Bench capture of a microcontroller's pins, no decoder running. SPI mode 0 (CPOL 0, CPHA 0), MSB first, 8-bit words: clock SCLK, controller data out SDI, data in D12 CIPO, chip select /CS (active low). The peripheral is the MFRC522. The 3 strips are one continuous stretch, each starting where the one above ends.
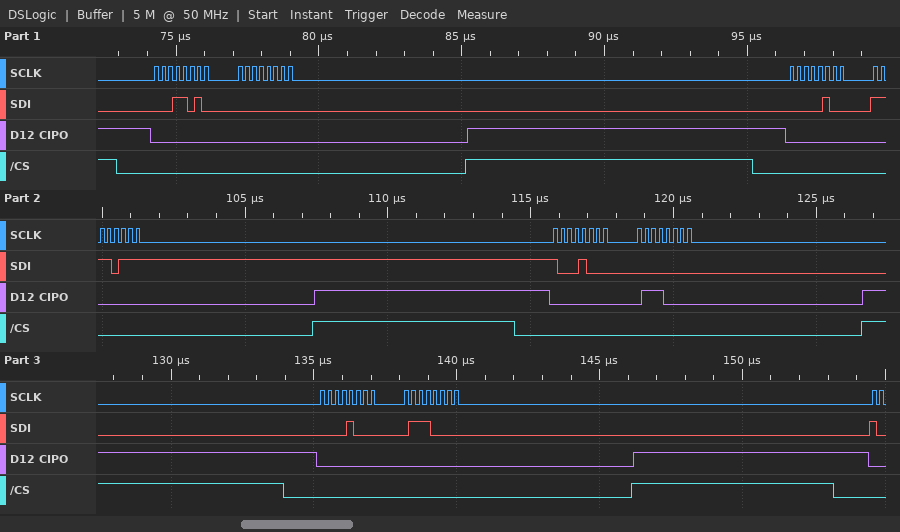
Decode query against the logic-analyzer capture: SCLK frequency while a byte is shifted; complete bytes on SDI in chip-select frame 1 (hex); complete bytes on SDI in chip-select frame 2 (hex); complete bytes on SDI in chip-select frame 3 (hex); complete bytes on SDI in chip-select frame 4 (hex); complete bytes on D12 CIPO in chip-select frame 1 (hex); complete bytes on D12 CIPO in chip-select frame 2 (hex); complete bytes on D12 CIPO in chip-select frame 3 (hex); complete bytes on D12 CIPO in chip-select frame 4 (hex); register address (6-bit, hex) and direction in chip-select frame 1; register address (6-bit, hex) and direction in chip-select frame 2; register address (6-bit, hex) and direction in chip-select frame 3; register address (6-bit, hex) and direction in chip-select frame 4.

4 MHz
1A 00
04 F7
88 00
08 70
00 00
00 00
00 70
00 00
0x0D write
0x02 write
0x04 read
0x04 write
